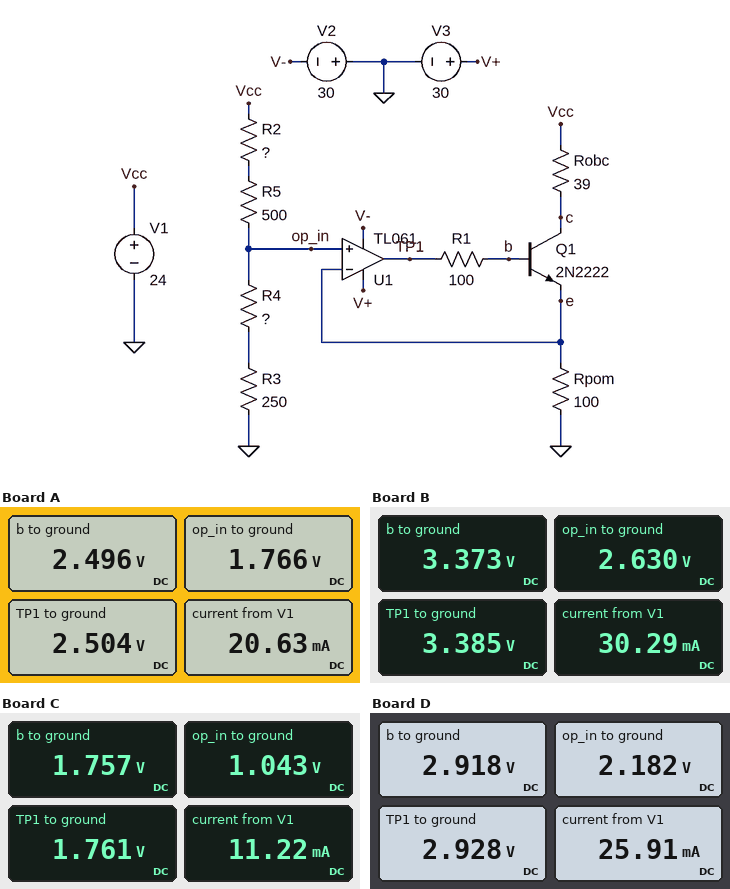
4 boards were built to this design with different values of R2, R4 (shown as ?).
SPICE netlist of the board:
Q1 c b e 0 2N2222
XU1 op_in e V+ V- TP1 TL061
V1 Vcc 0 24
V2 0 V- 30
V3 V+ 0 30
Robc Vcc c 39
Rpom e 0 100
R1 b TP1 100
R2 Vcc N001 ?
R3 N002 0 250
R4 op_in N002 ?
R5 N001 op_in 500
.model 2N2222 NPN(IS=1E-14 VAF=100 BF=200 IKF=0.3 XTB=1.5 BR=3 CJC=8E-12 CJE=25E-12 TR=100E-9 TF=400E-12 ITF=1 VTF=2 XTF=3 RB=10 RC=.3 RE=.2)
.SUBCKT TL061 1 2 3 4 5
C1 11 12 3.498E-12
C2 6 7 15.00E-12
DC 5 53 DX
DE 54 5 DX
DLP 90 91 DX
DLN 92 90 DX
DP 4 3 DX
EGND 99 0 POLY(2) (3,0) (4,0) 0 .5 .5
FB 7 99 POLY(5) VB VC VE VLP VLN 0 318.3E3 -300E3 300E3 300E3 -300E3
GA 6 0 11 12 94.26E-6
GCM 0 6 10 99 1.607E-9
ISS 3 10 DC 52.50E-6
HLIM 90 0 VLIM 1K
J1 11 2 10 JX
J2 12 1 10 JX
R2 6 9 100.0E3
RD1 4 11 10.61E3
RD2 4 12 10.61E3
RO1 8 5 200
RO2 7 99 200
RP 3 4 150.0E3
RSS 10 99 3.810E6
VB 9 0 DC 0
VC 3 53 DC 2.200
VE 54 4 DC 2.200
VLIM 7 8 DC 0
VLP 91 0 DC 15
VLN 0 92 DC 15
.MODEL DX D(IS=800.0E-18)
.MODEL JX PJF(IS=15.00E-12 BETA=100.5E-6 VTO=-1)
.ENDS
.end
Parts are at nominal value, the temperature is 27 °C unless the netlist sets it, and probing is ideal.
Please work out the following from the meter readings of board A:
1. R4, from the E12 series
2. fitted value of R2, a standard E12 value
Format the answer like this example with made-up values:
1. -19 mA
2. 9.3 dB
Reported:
1. 330 Ω
2. 6.8 kΩ
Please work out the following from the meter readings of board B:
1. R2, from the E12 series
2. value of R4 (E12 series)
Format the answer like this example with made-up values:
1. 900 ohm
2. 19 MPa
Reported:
1. 4.7 kΩ
2. 390 Ω
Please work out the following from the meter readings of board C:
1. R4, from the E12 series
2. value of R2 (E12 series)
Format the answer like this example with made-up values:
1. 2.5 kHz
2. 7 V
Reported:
1. 1 kΩ
2. 27 kΩ
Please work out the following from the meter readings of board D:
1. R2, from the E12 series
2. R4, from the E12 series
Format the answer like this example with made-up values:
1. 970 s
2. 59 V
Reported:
1. 4.7 kΩ
2. 270 Ω
